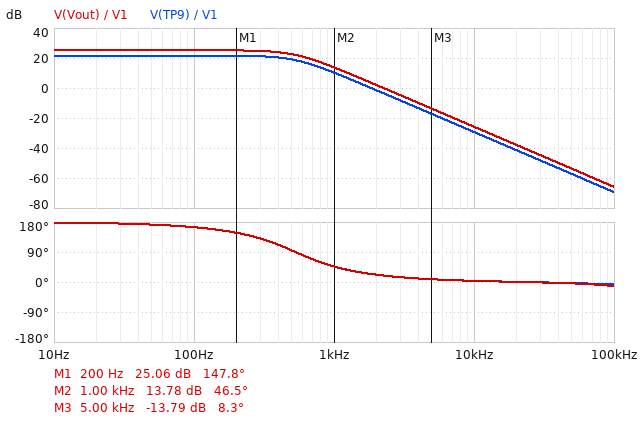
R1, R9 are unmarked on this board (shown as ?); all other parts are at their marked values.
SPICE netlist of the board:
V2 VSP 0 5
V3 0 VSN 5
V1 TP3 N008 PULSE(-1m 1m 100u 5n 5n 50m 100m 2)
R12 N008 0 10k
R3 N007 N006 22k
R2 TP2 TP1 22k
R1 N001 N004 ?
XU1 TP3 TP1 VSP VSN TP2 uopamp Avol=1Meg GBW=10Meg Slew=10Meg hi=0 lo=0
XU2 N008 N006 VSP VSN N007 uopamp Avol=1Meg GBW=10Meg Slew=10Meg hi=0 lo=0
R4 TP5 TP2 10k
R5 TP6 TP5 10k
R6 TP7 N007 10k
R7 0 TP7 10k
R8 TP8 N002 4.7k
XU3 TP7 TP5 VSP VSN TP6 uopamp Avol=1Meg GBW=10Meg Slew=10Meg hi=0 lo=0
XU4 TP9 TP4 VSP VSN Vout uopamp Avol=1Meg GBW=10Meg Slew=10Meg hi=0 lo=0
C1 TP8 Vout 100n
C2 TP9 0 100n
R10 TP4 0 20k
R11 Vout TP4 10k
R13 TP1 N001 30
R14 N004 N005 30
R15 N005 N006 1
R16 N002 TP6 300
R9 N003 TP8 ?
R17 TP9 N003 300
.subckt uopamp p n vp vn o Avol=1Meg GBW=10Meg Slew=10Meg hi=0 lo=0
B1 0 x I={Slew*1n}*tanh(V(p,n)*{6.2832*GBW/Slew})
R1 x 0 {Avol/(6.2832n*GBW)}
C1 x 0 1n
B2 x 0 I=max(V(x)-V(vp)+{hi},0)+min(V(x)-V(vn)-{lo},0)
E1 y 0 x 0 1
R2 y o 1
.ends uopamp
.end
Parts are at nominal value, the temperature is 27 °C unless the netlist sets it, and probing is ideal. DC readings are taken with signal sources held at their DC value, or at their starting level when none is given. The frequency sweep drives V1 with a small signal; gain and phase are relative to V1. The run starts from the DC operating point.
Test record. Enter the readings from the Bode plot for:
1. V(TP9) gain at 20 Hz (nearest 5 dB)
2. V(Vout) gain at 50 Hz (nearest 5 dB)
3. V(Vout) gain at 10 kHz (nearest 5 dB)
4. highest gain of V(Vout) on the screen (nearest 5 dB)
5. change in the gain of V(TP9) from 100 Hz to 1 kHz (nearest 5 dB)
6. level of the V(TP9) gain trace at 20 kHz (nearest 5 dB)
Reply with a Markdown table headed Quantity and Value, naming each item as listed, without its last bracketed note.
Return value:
| Quantity | Value |
|---|---|
| V(TP9) gain at 20 Hz | 20 dB |
| V(Vout) gain at 50 Hz | 25 dB |
| V(Vout) gain at 10 kHz | -25 dB |
| highest gain of V(Vout) on the screen | 25 dB |
| change in the gain of V(TP9) from 100 Hz to 1 kHz | -10 dB |
| level of the V(TP9) gain trace at 20 kHz | -40 dB |
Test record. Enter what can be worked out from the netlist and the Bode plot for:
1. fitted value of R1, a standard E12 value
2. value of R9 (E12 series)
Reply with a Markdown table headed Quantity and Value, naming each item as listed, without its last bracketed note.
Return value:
| Quantity | Value |
|---|---|
| fitted value of R1, a standard E12 value | 3.9 kΩ |
| value of R9 | 1.5 kΩ |
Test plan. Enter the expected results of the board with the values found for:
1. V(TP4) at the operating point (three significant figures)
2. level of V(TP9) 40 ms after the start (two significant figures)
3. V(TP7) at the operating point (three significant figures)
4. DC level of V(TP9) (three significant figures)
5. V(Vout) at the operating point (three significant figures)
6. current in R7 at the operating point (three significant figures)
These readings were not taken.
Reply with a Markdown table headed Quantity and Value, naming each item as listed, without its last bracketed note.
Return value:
| Quantity | Value |
|---|---|
| V(TP4) at the operating point | 12.1 mV |
| level of V(TP9) 40 ms after the start | -12 mV |
| V(TP7) at the operating point | 2.78 mV |
| DC level of V(TP9) | 12.1 mV |
| V(Vout) at the operating point | 18.2 mV |
| current in R7 at the operating point | 278 nA |
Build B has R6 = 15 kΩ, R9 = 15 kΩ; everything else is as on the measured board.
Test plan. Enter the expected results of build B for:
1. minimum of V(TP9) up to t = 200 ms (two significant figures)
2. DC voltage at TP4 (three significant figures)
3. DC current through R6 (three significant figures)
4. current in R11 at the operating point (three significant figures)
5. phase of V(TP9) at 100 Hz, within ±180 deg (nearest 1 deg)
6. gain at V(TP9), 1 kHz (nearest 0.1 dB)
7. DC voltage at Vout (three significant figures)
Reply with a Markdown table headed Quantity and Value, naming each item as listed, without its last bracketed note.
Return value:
| Quantity | Value |
|---|---|
| minimum of V(TP9) up to t = 200 ms | -11 mV |
| DC voltage at TP4 | 11.0 mV |
| DC current through R6 | 222 nA |
| current in R11 at the operating point | 550 nA |
| phase of V(TP9) at 100 Hz, within ±180 deg | 122 deg |
| gain at V(TP9), 1 kHz | -9.1 dB |
| DC voltage at Vout | 16.5 mV |
